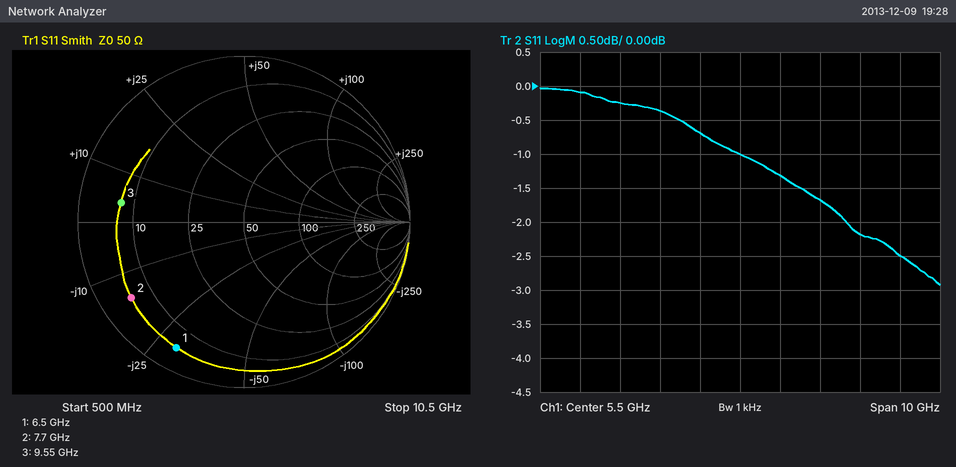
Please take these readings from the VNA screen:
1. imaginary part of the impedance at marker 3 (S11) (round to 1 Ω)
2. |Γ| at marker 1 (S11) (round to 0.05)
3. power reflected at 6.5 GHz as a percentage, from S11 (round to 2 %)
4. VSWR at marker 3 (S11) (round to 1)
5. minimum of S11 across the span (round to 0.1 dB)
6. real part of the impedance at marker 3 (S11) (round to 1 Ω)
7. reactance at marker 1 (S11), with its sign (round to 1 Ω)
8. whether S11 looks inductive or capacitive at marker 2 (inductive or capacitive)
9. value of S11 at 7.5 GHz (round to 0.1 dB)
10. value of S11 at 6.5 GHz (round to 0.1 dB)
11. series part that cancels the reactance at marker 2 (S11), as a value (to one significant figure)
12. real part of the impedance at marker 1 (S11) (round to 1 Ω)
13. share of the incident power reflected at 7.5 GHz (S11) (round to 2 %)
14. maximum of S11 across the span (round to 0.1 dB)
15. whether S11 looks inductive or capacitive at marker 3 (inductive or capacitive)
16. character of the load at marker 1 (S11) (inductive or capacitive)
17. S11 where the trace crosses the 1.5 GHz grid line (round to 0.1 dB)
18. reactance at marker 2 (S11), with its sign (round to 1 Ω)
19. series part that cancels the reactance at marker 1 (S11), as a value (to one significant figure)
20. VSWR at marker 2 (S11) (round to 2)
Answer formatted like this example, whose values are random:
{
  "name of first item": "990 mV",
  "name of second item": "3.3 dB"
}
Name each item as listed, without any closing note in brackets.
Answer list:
{
  "imaginary part of the impedance at marker 3 (S11)": "+4 Ω",
  "|Γ| at marker 1 (S11)": "0.85",
  "power reflected at 6.5 GHz as a percentage, from S11": "74 %",
  "VSWR at marker 3 (S11)": "7",
  "minimum of S11 across the span": "-2.9 dB",
  "real part of the impedance at marker 3 (S11)": "7 Ω",
  "reactance at marker 1 (S11), with its sign": "-30 Ω",
  "whether S11 looks inductive or capacitive at marker 2": "capacitive",
  "value of S11 at 7.5 GHz": "-1.7 dB",
  "value of S11 at 6.5 GHz": "-1.3 dB",
  "series part that cancels the reactance at marker 2 (S11), as a value": "300 pH",
  "real part of the impedance at marker 1 (S11)": "5 Ω",
  "share of the incident power reflected at 7.5 GHz (S11)": "68 %",
  "maximum of S11 across the span": "0.0 dB",
  "whether S11 looks inductive or capacitive at marker 3": "inductive",
  "character of the load at marker 1 (S11)": "capacitive",
  "S11 where the trace crosses the 1.5 GHz grid line": "-0.1 dB",
  "reactance at marker 2 (S11), with its sign": "-15 Ω",
  "series part that cancels the reactance at marker 1 (S11), as a value": "700 pH",
  "VSWR at marker 2 (S11)": "10"
}
